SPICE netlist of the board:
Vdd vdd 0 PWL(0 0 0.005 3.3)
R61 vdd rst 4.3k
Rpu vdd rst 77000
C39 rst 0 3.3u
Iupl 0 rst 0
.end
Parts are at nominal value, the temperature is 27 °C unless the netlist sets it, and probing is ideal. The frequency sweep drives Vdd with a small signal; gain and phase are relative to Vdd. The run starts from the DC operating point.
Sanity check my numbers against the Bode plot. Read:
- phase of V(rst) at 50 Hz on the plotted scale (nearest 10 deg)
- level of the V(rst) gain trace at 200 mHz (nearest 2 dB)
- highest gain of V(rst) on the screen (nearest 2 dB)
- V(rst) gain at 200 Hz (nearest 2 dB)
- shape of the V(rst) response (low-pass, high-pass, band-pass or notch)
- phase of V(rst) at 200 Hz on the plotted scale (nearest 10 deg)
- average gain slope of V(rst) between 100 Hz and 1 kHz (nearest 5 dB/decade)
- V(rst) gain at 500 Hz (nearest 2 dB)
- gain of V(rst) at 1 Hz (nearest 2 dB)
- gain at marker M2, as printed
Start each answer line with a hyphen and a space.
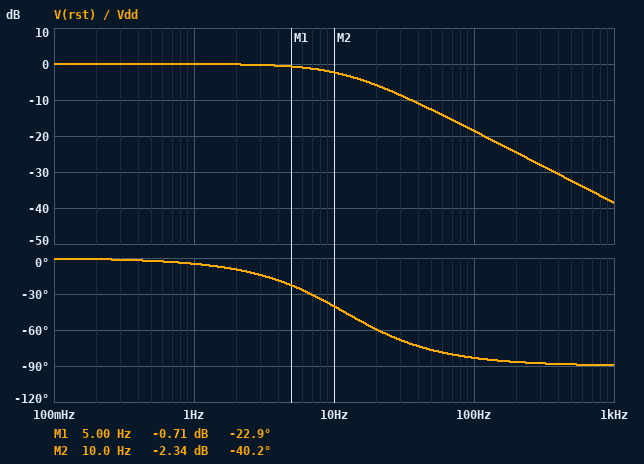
- -80 deg
- 0 dB
- 0 dB
- -24 dB
- low-pass
- -90 deg
- -20 dB/decade
- -32 dB
- 0 dB
- -2.34 dB
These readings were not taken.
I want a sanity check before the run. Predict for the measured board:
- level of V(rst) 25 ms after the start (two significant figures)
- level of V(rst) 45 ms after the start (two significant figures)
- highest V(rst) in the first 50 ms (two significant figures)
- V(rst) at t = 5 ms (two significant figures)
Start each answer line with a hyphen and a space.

- 2.7 V
- 3.2 V
- 3.2 V
- 540 mV
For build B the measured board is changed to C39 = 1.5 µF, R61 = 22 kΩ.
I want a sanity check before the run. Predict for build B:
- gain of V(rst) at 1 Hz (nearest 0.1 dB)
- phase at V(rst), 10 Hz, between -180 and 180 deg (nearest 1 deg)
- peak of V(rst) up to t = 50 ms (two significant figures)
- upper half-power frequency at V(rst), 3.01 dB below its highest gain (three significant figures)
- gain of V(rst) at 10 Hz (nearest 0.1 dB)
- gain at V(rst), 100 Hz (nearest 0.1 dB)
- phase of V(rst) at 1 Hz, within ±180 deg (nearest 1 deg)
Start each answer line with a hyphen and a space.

- -0.1 dB
- -58 deg
- 2.8 V
- 6.20 Hz
- -5.6 dB
- -24.2 dB
- -9 deg
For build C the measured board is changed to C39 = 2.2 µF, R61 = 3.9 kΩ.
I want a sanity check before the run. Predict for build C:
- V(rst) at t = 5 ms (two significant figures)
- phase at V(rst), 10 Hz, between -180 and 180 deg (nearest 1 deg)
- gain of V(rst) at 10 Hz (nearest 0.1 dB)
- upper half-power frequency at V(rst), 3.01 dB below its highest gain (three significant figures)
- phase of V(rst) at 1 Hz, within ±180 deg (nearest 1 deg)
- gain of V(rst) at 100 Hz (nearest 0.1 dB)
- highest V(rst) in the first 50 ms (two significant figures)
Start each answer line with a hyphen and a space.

- 830 mV
- -27 deg
- -1.0 dB
- 19.5 Hz
- -3 deg
- -14.4 dB
- 3.3 V
